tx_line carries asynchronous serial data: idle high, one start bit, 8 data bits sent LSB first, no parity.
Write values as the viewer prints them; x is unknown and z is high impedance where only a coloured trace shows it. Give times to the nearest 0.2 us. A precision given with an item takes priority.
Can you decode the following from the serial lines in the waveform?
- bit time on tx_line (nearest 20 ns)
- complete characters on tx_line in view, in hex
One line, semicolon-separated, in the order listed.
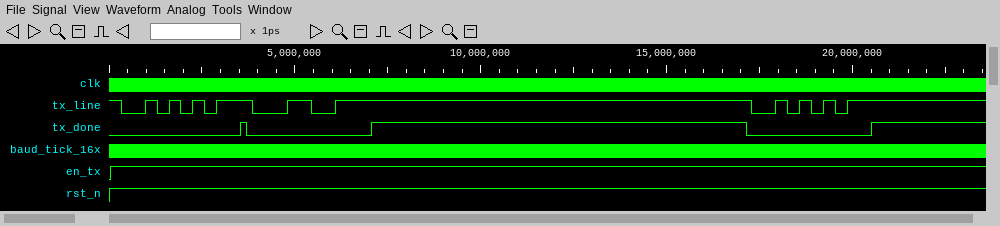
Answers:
320 ns; AA, CC, AA
